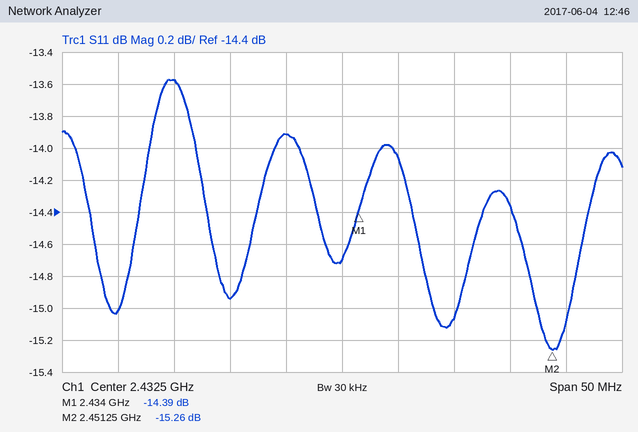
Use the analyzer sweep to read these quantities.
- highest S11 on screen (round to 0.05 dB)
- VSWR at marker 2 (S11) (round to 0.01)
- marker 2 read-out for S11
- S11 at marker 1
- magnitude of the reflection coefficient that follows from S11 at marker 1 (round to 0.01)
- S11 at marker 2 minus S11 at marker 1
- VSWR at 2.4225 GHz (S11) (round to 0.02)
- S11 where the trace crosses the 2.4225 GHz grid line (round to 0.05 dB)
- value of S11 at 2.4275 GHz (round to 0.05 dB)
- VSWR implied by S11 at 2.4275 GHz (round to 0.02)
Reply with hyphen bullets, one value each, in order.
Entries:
- -13.55 dB
- 1.42
- -15.26 dB
- -14.39 dB
- 0.19
- -0.87 dB
- 1.44
- -14.95 dB
- -13.90 dB
- 1.50
